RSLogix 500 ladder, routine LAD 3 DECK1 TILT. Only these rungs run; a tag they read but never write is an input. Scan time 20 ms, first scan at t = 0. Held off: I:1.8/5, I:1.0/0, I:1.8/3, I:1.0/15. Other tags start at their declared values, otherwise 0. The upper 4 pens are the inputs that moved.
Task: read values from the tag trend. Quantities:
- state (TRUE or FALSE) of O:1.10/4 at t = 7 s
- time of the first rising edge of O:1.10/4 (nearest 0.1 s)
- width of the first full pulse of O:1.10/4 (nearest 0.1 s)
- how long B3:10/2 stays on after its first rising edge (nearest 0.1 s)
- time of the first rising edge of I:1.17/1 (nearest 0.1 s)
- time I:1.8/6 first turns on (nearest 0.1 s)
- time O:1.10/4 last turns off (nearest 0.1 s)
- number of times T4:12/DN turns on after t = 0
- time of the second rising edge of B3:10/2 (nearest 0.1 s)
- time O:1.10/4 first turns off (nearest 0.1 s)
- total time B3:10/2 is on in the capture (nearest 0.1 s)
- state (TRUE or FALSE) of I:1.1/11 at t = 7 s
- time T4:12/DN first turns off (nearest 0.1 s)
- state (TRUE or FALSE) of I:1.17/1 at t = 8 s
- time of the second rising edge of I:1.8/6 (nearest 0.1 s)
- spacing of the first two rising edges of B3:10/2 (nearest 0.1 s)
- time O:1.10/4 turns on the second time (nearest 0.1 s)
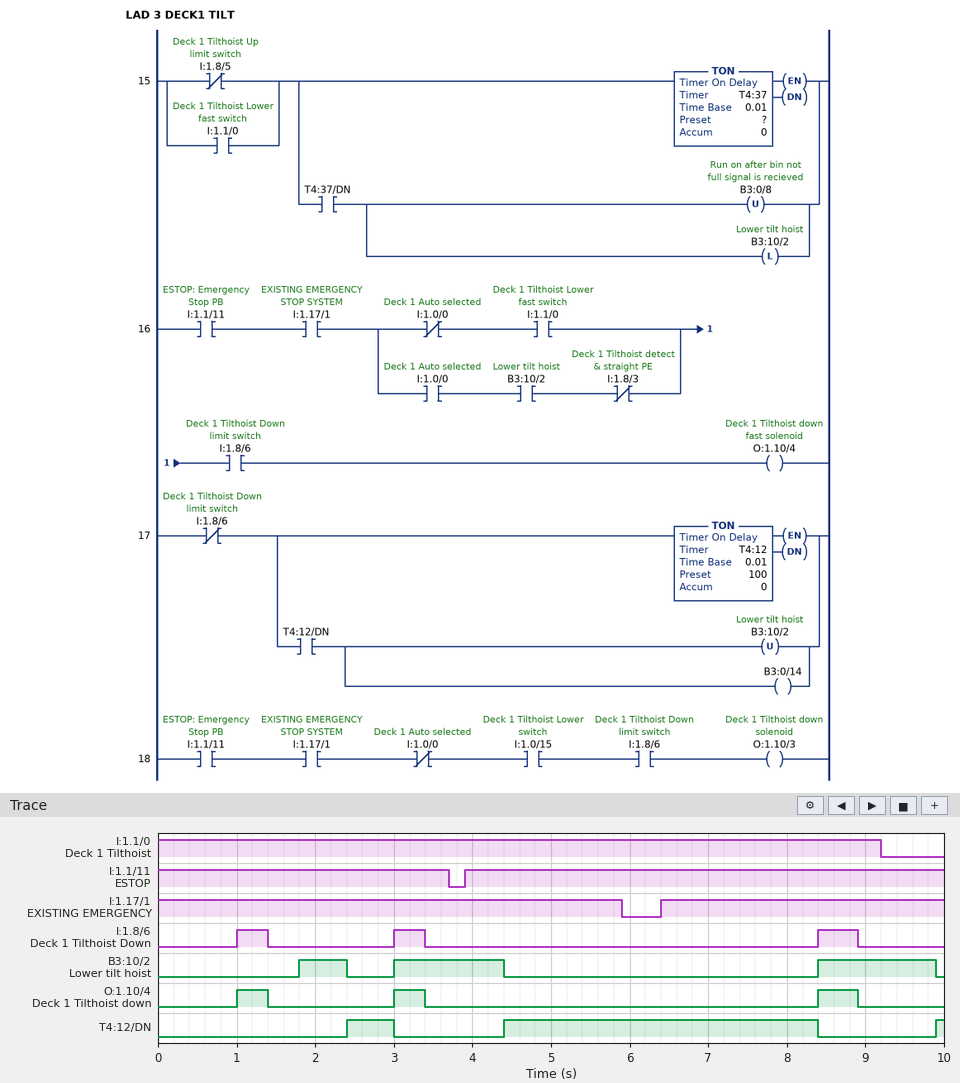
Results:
FALSE
1.0 s
0.4 s
0.6 s
6.4 s
1.0 s
8.9 s
3
3.0 s
1.4 s
3.5 s
TRUE
3.0 s
TRUE
3.0 s
1.2 s
3.0 s
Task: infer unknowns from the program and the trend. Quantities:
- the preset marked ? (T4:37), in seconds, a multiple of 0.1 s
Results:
1.8 s
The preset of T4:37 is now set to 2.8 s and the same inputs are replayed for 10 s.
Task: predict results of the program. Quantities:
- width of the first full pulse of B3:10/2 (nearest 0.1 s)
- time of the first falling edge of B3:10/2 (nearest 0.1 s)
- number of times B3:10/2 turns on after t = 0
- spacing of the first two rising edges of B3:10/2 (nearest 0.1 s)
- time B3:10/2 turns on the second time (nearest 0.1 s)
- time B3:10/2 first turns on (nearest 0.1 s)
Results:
1.4 s
4.4 s
2
5.4 s
8.4 s
3.0 s
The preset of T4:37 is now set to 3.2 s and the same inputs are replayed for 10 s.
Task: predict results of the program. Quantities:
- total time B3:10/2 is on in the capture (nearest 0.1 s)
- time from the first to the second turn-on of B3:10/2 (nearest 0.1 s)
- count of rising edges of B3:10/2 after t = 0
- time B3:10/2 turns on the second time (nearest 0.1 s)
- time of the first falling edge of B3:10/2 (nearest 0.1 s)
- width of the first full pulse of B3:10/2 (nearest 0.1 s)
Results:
2.7 s
5.2 s
2
8.4 s
4.4 s
1.2 s
